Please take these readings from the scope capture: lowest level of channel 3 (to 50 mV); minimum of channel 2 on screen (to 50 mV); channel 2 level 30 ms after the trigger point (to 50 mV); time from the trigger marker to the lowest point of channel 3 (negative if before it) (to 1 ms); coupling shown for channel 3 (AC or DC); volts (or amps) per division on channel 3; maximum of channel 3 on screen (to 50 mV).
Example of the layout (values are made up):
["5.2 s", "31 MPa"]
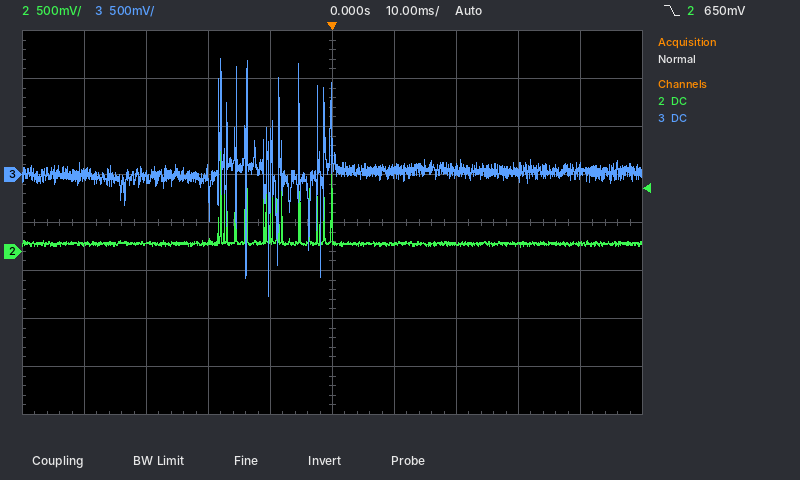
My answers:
["-1.25 V", "50 mV", "50 mV", "-10 ms", "DC", "500 mV", "1.20 V"]
